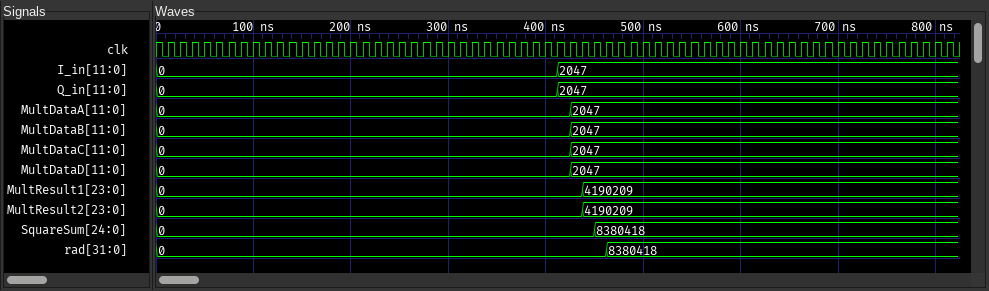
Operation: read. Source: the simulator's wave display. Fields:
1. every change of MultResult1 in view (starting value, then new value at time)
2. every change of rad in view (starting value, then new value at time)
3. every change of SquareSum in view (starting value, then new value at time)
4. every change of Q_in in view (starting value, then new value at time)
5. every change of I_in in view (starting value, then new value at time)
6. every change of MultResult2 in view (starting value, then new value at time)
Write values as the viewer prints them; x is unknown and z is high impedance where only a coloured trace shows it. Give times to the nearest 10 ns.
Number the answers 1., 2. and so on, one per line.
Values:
1. 0, 4190209 at 440 ns
2. 0, 8380418 at 460 ns
3. 0, 8380418 at 450 ns
4. 0, 2047 at 410 ns
5. 0, 2047 at 410 ns
6. 0, 4190209 at 440 ns
